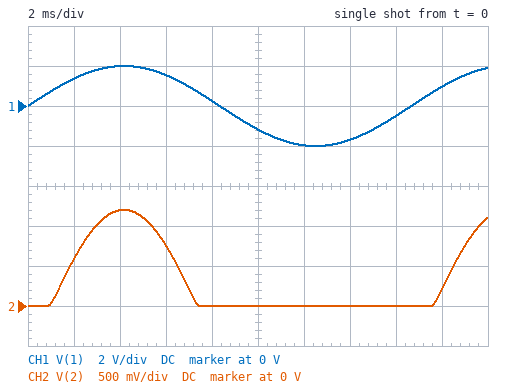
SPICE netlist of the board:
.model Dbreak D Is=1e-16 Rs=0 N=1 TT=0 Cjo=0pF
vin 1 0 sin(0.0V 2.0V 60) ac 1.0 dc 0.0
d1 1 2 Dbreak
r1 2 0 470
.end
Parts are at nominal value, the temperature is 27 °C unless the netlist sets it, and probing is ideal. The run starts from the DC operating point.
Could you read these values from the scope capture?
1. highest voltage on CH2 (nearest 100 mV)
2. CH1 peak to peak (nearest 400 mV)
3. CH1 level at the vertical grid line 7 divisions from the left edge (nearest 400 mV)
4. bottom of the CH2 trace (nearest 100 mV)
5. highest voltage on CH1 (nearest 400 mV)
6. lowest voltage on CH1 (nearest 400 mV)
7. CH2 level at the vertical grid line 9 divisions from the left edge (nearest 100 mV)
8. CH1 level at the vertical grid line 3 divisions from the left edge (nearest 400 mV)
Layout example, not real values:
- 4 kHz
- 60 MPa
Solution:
- 1.2 V
- 4.0 V
- -1.6 V
- 0 V
- 2.0 V
- -2.0 V
- 200 mV
- 1.6 V
